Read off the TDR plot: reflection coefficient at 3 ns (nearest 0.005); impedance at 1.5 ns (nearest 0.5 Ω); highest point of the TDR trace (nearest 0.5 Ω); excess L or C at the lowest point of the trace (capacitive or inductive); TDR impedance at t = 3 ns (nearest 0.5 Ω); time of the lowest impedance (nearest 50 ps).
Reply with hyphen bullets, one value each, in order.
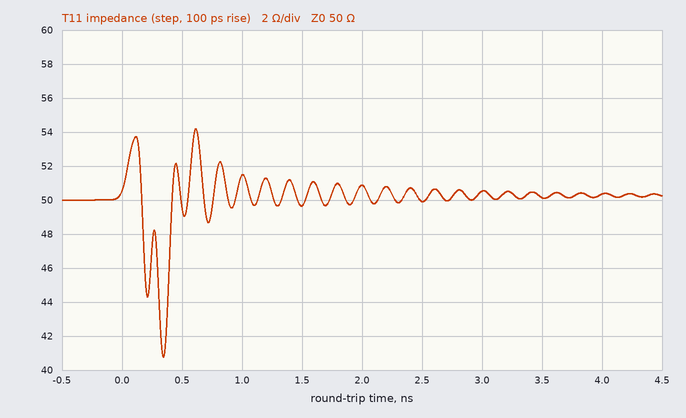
- +0.005
- 49.5 Ω
- 54.0 Ω
- capacitive
- 50.5 Ω
- 350 ps
